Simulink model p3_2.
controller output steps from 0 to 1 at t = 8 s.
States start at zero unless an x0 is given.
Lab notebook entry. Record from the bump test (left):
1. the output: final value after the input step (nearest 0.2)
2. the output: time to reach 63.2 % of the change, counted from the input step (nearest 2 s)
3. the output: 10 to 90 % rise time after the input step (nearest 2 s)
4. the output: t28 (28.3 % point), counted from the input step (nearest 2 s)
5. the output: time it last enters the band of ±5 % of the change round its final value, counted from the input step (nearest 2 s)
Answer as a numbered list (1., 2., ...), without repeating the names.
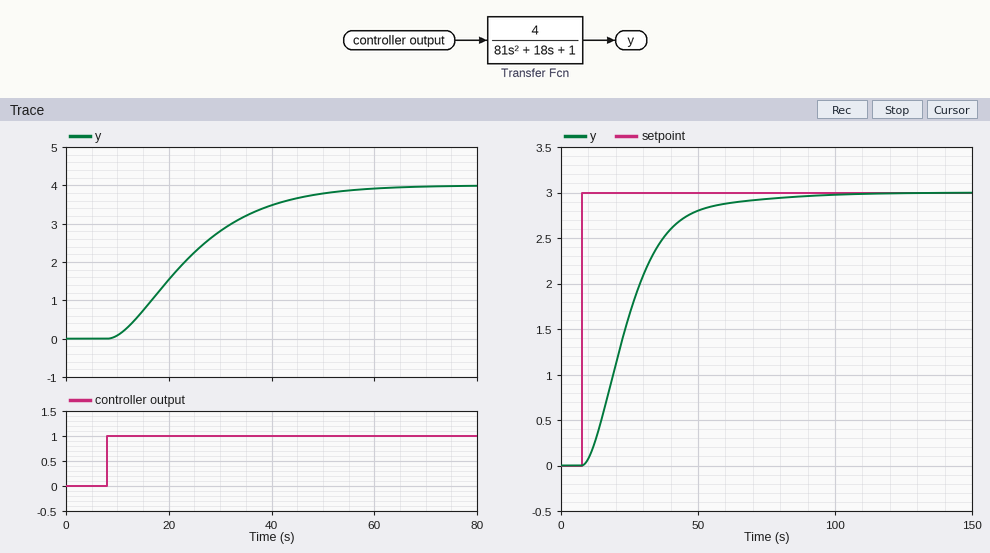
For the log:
1. 4.0
2. 20 s
3. 30 s
4. 10 s
5. 42 s
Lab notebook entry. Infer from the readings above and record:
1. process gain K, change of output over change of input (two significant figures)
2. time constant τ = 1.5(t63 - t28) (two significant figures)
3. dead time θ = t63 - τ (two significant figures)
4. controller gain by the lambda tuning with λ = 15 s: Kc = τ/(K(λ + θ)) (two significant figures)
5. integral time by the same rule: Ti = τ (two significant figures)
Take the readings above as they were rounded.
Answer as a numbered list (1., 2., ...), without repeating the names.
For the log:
1. 4.0
2. 15 s
3. 5.0 s
4. 0.19
5. 15 s
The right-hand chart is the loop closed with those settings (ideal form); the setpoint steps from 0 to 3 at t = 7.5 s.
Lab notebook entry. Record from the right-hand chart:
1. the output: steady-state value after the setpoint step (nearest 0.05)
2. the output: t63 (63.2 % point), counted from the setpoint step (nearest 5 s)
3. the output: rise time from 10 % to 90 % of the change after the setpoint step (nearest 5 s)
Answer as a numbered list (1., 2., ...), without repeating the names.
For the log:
1. 3.00
2. 20 s
3. 30 s
